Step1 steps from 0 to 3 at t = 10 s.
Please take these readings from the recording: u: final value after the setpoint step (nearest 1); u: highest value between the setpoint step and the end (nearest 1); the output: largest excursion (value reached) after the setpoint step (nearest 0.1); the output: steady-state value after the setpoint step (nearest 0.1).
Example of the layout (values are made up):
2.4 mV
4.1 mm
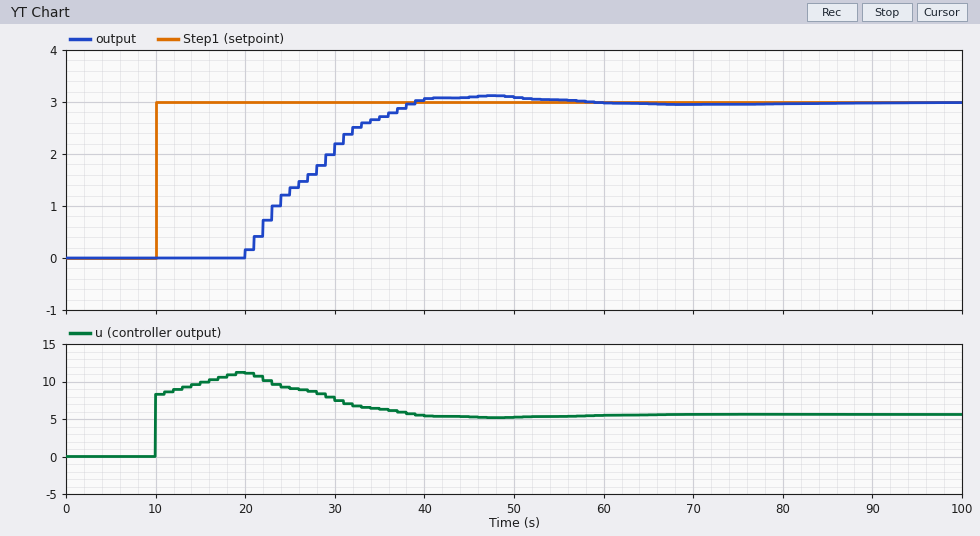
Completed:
6
11
3.1
3.0
